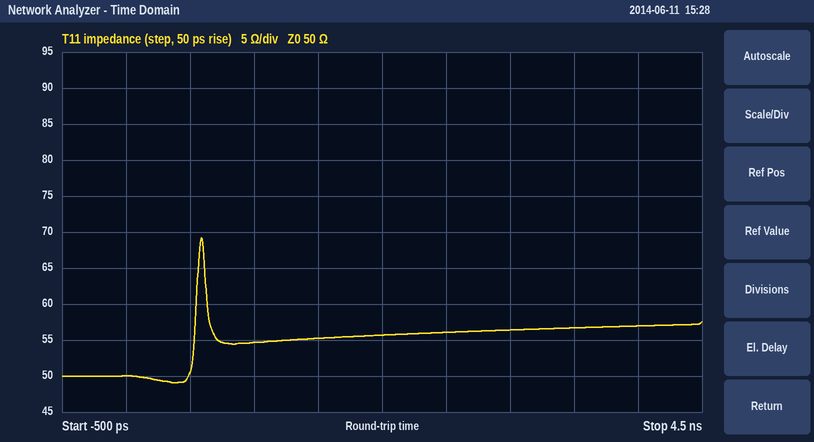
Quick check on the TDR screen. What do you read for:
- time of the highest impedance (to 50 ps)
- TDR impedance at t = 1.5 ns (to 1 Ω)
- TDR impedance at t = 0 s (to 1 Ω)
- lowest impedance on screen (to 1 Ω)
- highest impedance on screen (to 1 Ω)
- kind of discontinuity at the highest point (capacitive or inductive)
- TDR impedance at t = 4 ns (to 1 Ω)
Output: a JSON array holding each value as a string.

["600 ps", "55 Ω", "50 Ω", "49 Ω", "69 Ω", "inductive", "57 Ω"]
